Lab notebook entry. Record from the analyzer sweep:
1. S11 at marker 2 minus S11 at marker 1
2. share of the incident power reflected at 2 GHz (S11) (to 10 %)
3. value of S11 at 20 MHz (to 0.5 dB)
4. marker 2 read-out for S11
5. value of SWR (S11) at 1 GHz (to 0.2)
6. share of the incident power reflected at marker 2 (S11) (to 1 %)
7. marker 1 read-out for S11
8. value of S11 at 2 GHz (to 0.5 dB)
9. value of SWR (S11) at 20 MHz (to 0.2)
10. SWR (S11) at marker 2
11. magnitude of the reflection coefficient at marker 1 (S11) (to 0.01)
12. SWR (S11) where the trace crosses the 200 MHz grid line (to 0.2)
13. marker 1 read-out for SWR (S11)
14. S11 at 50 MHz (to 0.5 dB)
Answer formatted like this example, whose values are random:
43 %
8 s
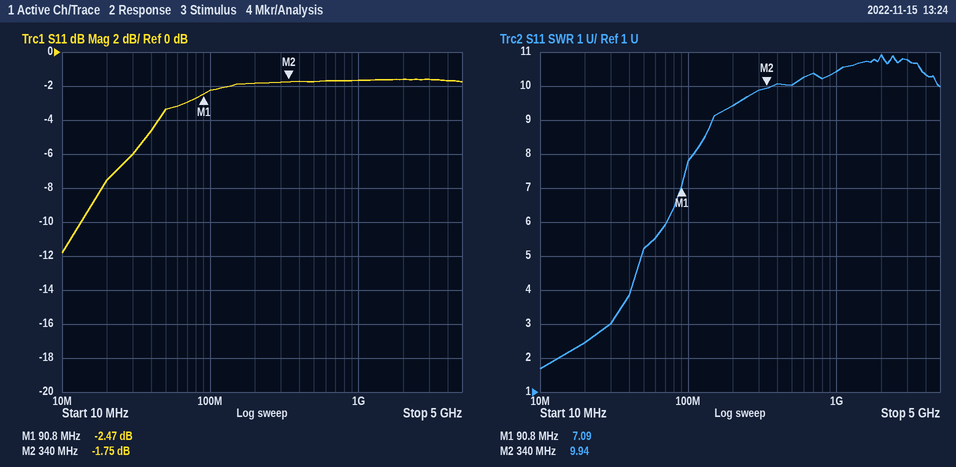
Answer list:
0.72 dB
70 %
-7.5 dB
-1.75 dB
10.4
67 %
-2.47 dB
-1.5 dB
2.4
9.94
0.75
9.4
7.09
-3.5 dB
